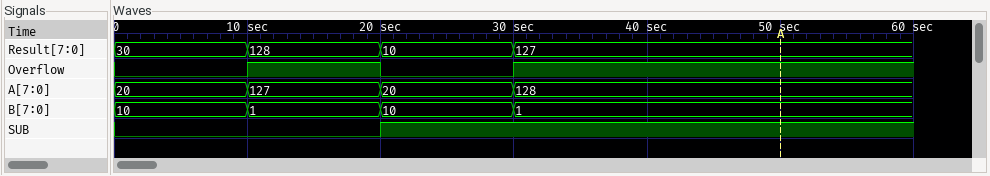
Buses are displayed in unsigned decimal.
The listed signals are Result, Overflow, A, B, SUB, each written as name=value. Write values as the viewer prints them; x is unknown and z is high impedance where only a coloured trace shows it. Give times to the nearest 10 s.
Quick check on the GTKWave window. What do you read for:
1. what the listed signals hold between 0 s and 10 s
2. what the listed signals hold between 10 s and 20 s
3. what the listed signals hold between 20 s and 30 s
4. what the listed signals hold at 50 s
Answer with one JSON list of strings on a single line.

["Result=30, Overflow=0, A=20, B=10, SUB=0", "Result=128, Overflow=1, A=127, B=1, SUB=0", "Result=10, Overflow=0, A=20, B=10, SUB=1", "Result=127, Overflow=1, A=128, B=1, SUB=1"]
